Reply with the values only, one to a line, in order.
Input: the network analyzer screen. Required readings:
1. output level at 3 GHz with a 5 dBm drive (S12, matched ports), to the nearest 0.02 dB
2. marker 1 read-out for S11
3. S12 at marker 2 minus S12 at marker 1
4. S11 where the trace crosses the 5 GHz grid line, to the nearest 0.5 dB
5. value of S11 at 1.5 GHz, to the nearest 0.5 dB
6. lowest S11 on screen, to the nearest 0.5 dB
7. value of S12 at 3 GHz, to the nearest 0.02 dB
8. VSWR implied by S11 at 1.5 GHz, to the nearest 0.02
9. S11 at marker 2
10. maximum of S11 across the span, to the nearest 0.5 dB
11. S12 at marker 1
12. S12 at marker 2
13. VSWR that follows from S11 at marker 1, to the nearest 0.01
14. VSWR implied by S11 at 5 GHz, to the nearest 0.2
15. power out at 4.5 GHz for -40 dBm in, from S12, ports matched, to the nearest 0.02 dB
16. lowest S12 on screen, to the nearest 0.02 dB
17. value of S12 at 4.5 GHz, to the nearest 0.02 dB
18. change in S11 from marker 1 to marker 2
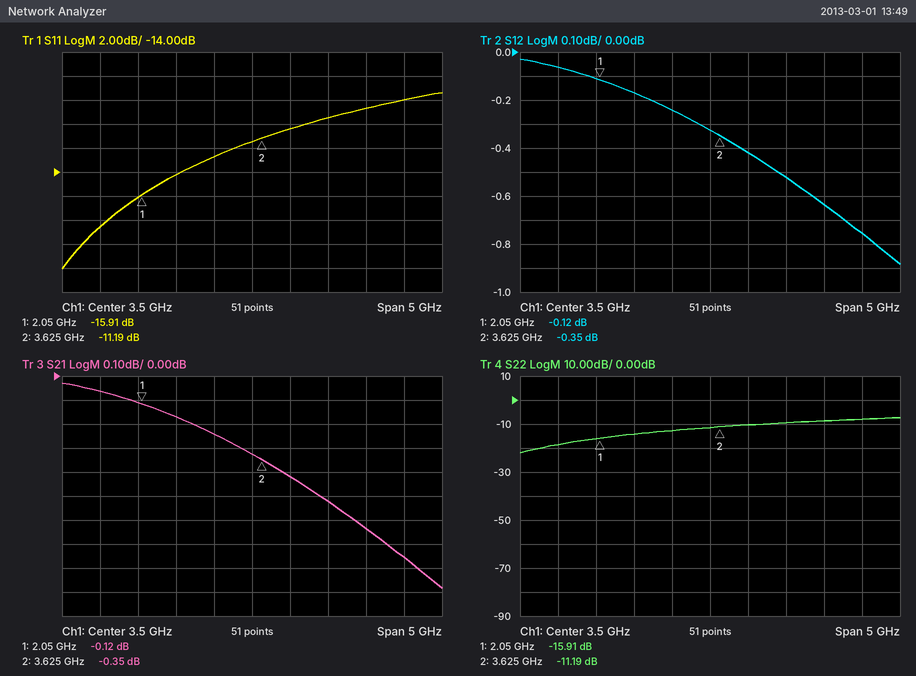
4.76 dBm
-15.91 dB
-0.23 dB
-8.5 dB
-18.5 dB
-22.0 dB
-0.24 dB
1.26
-11.19 dB
-7.5 dB
-0.12 dB
-0.35 dB
1.38
2.2
-40.52 dBm
-0.88 dB
-0.52 dB
4.72 dB
